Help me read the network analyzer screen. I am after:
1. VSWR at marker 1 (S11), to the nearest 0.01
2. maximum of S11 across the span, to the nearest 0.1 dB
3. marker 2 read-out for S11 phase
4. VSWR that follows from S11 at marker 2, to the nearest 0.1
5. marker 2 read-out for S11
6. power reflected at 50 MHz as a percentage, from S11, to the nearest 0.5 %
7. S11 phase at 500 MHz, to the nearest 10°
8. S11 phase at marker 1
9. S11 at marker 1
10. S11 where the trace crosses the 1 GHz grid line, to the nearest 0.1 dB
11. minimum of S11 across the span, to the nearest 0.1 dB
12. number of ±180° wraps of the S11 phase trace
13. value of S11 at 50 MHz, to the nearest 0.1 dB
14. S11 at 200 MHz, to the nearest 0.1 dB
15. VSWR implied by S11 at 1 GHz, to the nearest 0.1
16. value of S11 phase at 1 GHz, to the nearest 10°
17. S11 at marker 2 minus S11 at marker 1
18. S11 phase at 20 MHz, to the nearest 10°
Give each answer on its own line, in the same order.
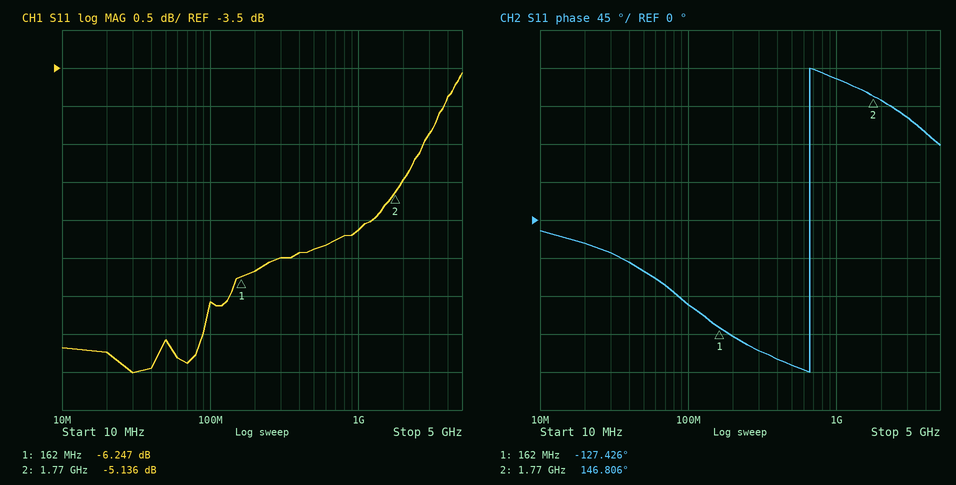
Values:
2.90
-3.6 dB
146.806°
3.5
-5.136 dB
19.5 %
-170°
-127.426°
-6.247 dB
-5.6 dB
-7.5 dB
1
-7.1 dB
-6.2 dB
3.2
170°
1.111 dB
-30°
